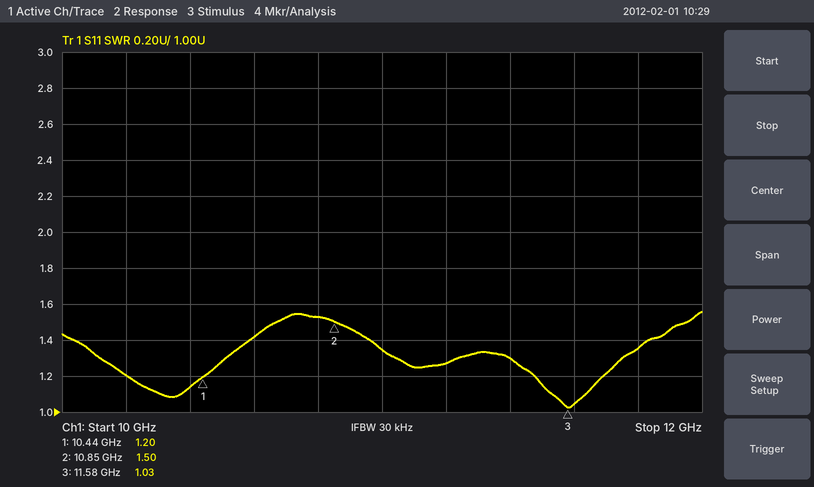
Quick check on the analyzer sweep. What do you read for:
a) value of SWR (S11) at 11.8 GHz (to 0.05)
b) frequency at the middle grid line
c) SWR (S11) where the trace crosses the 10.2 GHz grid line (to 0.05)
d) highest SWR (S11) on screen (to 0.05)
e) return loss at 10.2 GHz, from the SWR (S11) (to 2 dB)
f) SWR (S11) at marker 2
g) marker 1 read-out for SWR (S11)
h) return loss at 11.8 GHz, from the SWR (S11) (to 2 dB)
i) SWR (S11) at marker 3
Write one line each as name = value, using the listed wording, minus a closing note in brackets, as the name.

value of SWR (S11) at 11.8 GHz = 1.35
frequency at the middle grid line = 11 GHz
SWR (S11) where the trace crosses the 10.2 GHz grid line = 1.20
highest SWR (S11) on screen = 1.55
return loss at 10.2 GHz, from the SWR (S11) = 20 dB
SWR (S11) at marker 2 = 1.50
marker 1 read-out for SWR = 1.20
return loss at 11.8 GHz, from the SWR (S11) = 16 dB
SWR (S11) at marker 3 = 1.03
